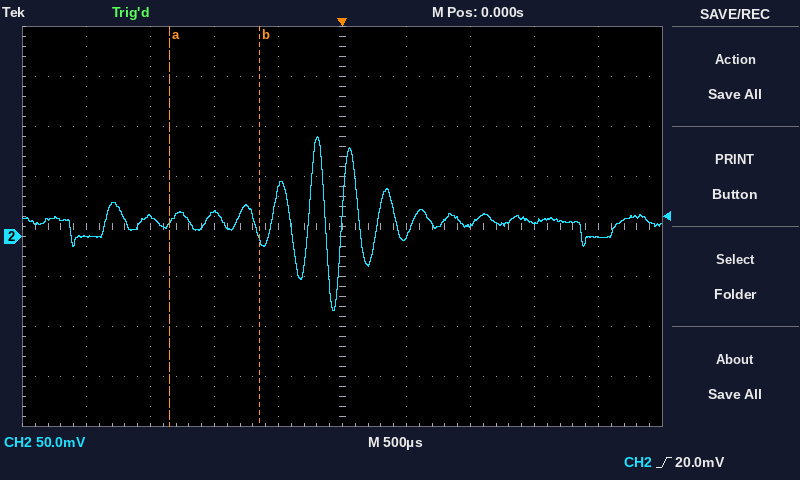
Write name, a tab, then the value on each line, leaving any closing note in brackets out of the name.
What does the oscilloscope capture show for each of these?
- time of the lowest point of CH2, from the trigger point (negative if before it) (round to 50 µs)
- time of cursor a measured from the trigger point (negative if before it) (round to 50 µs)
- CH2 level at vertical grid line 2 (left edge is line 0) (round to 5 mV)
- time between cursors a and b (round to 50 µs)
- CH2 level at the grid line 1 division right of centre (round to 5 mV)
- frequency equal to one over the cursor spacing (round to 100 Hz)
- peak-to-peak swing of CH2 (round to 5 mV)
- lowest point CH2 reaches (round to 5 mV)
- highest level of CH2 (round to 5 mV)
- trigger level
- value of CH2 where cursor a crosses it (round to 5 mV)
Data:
time of the lowest point of CH2, from the trigger point (negative if before it)	-50 µs
time of cursor a measured from the trigger point (negative if before it)	-1.35 ms
CH2 level at vertical grid line 2 (left edge is line 0)	20 mV
time between cursors a and b	700 µs
CH2 level at the grid line 1 division right of centre	0 mV
frequency equal to one over the cursor spacing	1.4 kHz
peak-to-peak swing of CH2	175 mV
lowest point CH2 reaches	-75 mV
highest level of CH2	100 mV
trigger level	20.0 mV
value of CH2 where cursor a crosses it	15 mV
